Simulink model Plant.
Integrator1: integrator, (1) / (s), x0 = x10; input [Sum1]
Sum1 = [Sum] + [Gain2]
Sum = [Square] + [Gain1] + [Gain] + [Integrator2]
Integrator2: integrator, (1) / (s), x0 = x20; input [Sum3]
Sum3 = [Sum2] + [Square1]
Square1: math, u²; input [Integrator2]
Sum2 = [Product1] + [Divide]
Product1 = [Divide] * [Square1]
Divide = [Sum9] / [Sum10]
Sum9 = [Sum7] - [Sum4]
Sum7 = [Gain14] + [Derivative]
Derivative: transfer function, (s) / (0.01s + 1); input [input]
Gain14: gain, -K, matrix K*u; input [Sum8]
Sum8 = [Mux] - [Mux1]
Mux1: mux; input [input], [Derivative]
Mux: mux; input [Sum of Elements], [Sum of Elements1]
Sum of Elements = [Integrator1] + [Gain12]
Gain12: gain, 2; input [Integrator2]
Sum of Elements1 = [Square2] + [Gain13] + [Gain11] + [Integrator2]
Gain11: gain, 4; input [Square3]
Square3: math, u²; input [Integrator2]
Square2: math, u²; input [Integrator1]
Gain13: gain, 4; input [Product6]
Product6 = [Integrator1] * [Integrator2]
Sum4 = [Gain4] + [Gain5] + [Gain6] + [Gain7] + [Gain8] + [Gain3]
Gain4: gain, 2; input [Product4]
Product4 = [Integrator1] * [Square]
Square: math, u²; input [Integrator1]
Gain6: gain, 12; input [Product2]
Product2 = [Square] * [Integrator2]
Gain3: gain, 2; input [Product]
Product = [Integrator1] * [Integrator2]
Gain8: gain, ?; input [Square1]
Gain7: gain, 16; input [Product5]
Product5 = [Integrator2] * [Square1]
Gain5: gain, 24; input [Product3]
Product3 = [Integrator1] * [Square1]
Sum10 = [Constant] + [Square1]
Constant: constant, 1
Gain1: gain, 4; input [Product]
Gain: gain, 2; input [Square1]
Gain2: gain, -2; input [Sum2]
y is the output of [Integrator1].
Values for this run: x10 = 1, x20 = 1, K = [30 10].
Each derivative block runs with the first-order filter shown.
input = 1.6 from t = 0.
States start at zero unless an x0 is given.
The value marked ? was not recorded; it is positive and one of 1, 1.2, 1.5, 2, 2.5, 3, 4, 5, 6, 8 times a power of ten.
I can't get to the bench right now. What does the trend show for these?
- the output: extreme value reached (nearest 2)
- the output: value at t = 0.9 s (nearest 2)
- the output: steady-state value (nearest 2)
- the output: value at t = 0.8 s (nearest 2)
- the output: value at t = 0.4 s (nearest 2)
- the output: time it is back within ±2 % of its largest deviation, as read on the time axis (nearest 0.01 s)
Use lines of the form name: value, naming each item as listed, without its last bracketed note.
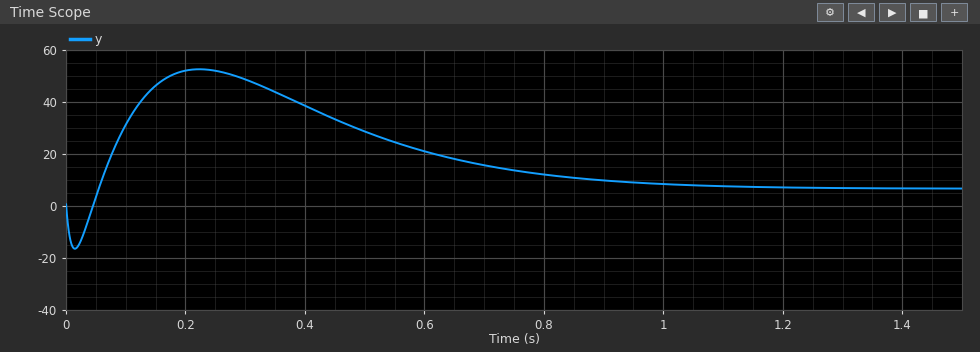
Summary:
the output: extreme value reached: 52
the output: value at t = 0.9 s: 10
the output: steady-state value: 6
the output: value at t = 0.8 s: 12
the output: value at t = 0.4 s: 38
the output: time it is back within ±2 % of its largest deviation, as read on the time axis: 1.08 s
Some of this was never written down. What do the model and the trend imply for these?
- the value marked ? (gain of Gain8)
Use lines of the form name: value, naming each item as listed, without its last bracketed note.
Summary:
the value marked ?: 5
